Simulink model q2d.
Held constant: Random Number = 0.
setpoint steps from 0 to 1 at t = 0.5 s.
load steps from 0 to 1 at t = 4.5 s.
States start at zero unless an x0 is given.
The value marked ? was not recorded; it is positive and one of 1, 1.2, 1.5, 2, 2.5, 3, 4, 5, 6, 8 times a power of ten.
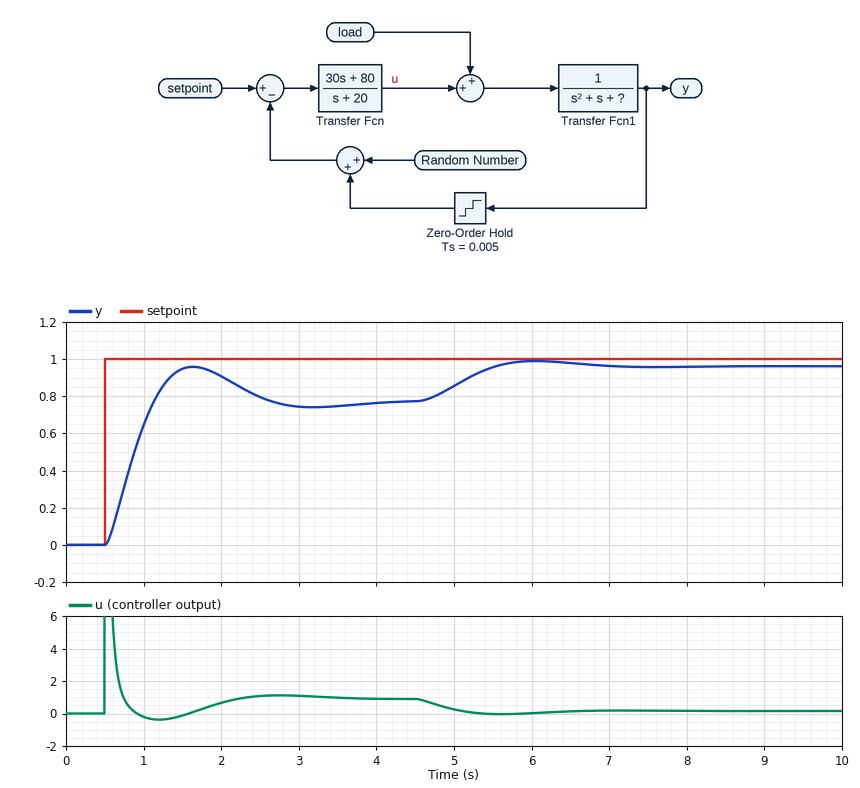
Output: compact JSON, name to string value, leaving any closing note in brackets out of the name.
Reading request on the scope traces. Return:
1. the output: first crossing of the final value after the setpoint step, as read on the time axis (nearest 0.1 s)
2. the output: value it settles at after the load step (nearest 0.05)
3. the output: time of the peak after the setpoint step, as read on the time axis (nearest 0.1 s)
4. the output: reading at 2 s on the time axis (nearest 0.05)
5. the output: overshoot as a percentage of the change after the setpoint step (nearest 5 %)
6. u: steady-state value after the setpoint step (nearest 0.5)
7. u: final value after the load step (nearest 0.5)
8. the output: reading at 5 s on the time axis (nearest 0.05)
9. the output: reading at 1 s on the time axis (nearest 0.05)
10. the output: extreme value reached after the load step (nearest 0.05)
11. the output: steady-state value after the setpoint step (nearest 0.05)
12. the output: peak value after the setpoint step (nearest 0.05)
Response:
{"the output: first crossing of the final value after the setpoint step, as read on the time axis": "1.1 s", "the output: value it settles at after the load step": "0.95", "the output: time of the peak after the setpoint step, as read on the time axis": "1.6 s", "the output: reading at 2 s on the time axis": "0.90", "the output: overshoot as a percentage of the change after the setpoint step": "25 %", "u: steady-state value after the setpoint step": "1.0", "u: final value after the load step": "0.0", "the output: reading at 5 s on the time axis": "0.85", "the output: reading at 1 s on the time axis": "0.65", "the output: extreme value reached after the load step": "1.00", "the output: steady-state value after the setpoint step": "0.75", "the output: peak value after the setpoint step": "0.95"}
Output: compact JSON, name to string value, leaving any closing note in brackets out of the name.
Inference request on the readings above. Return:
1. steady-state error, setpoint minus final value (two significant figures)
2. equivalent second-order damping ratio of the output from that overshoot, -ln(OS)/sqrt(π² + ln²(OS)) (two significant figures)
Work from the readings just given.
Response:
{"steady-state error, setpoint minus final value": "0.25", "equivalent second-order damping ratio of the output from that overshoot, -ln(OS)/sqrt(π² + ln²(OS))": "0.40"}
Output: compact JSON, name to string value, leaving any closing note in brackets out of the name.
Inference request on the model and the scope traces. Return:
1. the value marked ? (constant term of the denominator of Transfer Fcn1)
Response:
{"the value marked ?": "1.2"}
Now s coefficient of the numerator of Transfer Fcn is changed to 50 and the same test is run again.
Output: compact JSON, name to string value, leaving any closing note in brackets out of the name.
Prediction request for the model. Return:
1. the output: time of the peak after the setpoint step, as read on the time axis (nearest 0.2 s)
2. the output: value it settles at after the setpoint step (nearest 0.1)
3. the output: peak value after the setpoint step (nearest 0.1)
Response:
{"the output: time of the peak after the setpoint step, as read on the time axis": "1.4 s", "the output: value it settles at after the setpoint step": "0.8", "the output: peak value after the setpoint step": "0.9"}
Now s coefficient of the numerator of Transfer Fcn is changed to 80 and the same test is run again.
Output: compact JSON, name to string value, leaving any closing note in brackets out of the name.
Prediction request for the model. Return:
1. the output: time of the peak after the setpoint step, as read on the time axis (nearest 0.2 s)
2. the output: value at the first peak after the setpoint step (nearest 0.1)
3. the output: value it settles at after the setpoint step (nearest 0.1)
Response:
{"the output: time of the peak after the setpoint step, as read on the time axis": "1.2 s", "the output: value at the first peak after the setpoint step": "0.9", "the output: value it settles at after the setpoint step": "0.8"}
